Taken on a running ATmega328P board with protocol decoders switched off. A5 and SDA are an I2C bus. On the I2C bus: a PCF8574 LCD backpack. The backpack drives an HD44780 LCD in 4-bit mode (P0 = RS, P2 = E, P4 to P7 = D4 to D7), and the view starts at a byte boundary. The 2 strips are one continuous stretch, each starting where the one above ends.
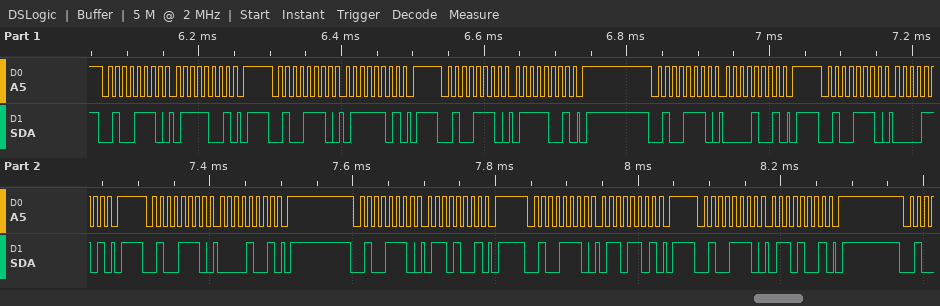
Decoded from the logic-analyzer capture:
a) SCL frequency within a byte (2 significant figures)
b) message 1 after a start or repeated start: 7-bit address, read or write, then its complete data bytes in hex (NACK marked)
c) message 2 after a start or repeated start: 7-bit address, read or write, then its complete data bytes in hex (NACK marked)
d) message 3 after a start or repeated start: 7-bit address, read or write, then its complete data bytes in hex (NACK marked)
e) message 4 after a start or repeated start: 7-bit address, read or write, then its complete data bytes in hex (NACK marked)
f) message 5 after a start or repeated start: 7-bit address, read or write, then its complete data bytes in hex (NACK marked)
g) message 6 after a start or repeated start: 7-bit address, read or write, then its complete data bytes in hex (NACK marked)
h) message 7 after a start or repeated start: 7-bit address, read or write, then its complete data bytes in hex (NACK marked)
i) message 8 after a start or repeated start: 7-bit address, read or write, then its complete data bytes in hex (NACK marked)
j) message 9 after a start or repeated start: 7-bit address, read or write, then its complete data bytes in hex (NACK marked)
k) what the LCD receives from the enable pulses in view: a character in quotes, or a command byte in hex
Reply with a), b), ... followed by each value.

a) 100 kHz
b) 0x27 write: 79
c) 0x27 write: 7D
d) 0x27 write: 79
e) 0x27 write: 09
f) 0x27 write: 0D
g) 0x27 write: 09
h) 0x27 write: 69
i) 0x27 write: 6D
j) 0x27 write: 69
k) 'p'
